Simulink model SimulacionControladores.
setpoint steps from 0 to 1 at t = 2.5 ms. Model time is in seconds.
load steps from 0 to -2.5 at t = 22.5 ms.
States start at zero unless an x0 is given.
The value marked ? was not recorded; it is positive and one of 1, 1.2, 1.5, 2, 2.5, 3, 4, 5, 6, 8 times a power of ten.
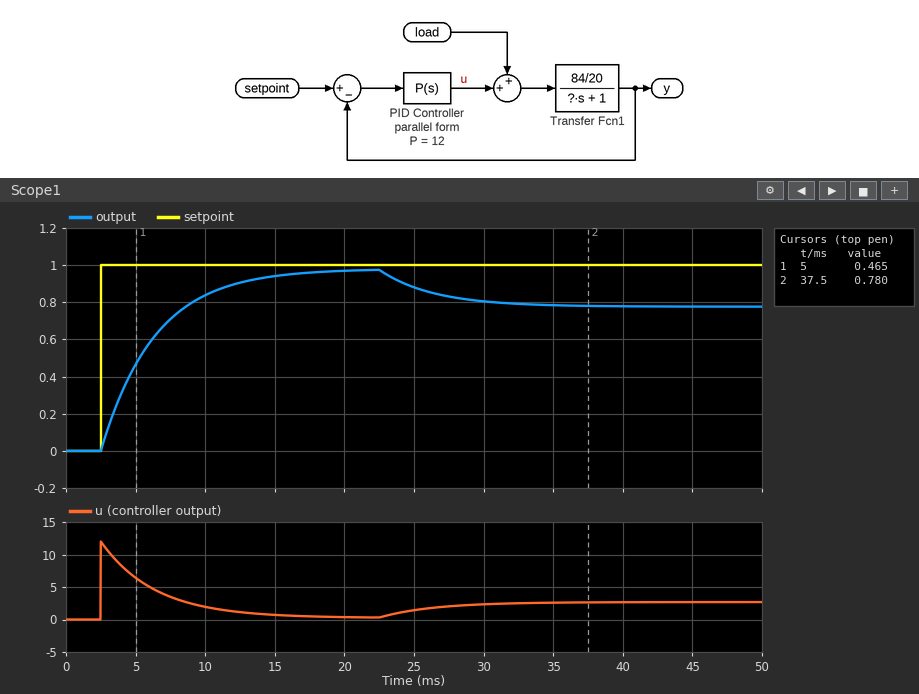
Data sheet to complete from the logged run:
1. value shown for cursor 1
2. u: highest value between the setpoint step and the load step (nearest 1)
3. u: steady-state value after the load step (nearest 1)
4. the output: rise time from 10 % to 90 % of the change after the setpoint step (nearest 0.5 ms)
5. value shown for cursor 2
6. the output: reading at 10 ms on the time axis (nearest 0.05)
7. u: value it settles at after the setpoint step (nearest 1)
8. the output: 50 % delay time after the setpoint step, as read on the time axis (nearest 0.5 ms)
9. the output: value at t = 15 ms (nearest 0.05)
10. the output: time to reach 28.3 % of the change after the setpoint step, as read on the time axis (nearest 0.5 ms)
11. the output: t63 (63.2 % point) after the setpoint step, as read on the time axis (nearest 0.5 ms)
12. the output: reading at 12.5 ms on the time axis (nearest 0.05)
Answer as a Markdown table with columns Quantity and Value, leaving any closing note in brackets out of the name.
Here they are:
| Quantity | Value |
|---|---|
| value shown for cursor 1 | 0.465 |
| u: highest value between the setpoint step and the load step | 12 |
| u: steady-state value after the load step | 3 |
| the output: rise time from 10 % to 90 % of the change after the setpoint step | 8.5 ms |
| value shown for cursor 2 | 0.780 |
| the output: reading at 10 ms on the time axis | 0.85 |
| u: value it settles at after the setpoint step | 0 |
| the output: 50 % delay time after the setpoint step, as read on the time axis | 5.0 ms |
| the output: value at t = 15 ms | 0.95 |
| the output: time to reach 28.3 % of the change after the setpoint step, as read on the time axis | 4.0 ms |
| the output: t63 (63.2 % point) after the setpoint step, as read on the time axis | 6.5 ms |
| the output: reading at 12.5 ms on the time axis | 0.90 |
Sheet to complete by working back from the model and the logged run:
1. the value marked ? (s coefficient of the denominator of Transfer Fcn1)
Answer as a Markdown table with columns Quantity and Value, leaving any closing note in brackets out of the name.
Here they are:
| Quantity | Value |
|---|---|
| the value marked ? | 0.2 |
